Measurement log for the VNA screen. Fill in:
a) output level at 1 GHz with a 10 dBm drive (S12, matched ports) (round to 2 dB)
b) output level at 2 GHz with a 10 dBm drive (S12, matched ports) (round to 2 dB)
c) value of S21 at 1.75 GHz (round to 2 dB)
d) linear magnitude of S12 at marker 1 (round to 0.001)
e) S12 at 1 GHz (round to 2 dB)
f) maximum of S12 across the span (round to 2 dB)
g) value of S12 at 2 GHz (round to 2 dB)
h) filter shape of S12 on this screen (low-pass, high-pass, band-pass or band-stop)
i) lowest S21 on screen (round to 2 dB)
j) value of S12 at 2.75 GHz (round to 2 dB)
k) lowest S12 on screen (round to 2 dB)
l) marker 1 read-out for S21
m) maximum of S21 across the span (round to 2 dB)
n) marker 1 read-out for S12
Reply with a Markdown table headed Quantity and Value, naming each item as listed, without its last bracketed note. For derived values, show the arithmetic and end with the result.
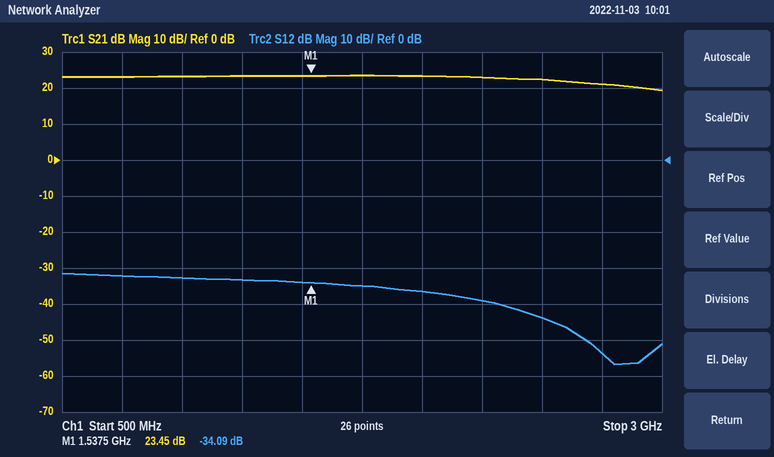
| Quantity | Value |
|---|---|
| output level at 1 GHz with a 10 dBm drive (S12, matched ports) | 10 dBm + (-32 dB) = -22 dBm |
| output level at 2 GHz with a 10 dBm drive (S12, matched ports) | 10 dBm + (-36 dB) = -26 dBm |
| value of S21 at 1.75 GHz | 24 dB |
| linear magnitude of S12 at marker 1 | 10^(-34.09/20) ≈ 0.020 |
| S12 at 1 GHz | -32 dB |
| maximum of S12 across the span | -32 dB |
| value of S12 at 2 GHz | -36 dB |
| filter shape of S12 on this screen | low-pass |
| lowest S21 on screen | 20 dB |
| value of S12 at 2.75 GHz | -54 dB |
| lowest S12 on screen | -56 dB |
| marker 1 read-out for S21 | 23.45 dB |
| maximum of S21 across the span | 24 dB |
| marker 1 read-out for S12 | -34.09 dB |
